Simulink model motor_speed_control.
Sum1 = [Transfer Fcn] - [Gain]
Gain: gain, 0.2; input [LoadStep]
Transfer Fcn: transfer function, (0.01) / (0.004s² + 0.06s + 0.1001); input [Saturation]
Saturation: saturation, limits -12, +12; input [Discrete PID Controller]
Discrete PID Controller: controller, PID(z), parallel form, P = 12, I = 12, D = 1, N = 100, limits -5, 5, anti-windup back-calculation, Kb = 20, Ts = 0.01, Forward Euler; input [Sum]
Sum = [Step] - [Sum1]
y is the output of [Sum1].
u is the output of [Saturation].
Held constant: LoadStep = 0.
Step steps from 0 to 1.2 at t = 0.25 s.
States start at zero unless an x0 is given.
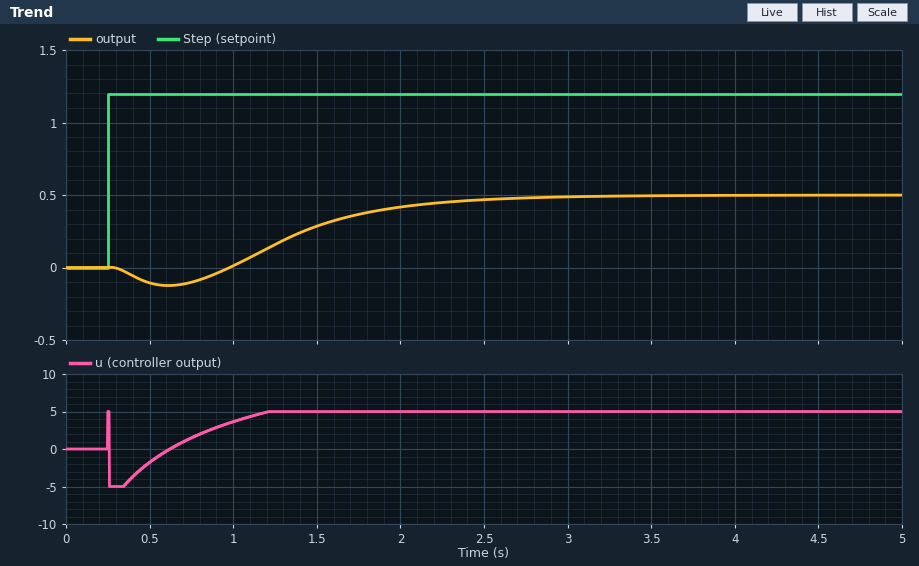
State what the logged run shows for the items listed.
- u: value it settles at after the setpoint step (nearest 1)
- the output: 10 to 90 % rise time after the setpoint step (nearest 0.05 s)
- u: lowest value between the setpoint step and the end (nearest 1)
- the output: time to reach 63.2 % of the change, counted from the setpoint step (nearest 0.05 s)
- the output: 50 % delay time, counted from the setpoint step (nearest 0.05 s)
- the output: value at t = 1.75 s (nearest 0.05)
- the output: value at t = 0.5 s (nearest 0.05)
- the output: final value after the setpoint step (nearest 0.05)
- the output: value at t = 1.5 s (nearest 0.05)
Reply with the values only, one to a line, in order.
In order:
5
1.20 s
-5
1.35 s
1.15 s
0.35
-0.10
0.50
0.30
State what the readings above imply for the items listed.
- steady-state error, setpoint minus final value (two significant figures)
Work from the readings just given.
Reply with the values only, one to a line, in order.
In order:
0.70
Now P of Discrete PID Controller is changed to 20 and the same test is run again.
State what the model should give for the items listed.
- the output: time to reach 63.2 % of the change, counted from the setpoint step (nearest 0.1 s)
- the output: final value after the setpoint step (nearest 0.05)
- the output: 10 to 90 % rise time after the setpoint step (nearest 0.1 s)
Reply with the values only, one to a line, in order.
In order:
1.2 s
0.50
1.3 s
